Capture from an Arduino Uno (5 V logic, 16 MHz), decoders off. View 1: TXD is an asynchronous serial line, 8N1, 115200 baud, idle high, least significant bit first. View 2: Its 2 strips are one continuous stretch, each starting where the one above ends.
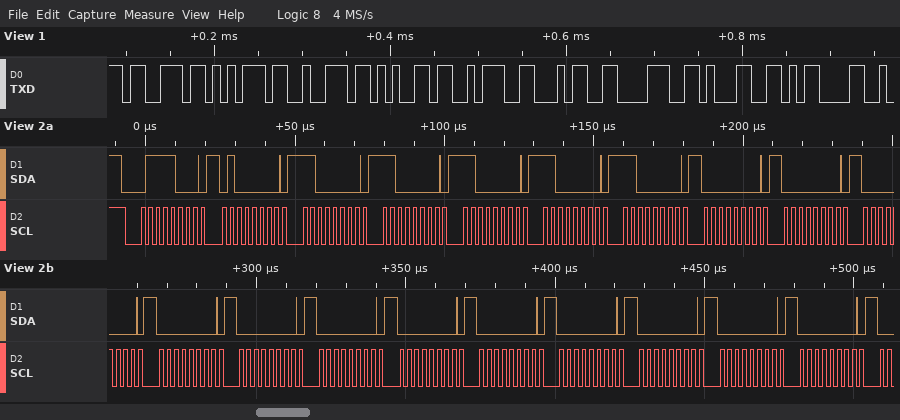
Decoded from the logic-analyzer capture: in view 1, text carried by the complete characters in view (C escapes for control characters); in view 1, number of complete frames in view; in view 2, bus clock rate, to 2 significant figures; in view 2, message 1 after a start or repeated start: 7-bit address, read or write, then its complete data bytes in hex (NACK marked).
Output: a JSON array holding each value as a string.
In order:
["\"sure:481\\r\"", "9", "400 kHz", "0x3C write: 40 C0 C0 C0 C0 C0 00 00 00 00 00 00 00 00 00 00 00 00"]
